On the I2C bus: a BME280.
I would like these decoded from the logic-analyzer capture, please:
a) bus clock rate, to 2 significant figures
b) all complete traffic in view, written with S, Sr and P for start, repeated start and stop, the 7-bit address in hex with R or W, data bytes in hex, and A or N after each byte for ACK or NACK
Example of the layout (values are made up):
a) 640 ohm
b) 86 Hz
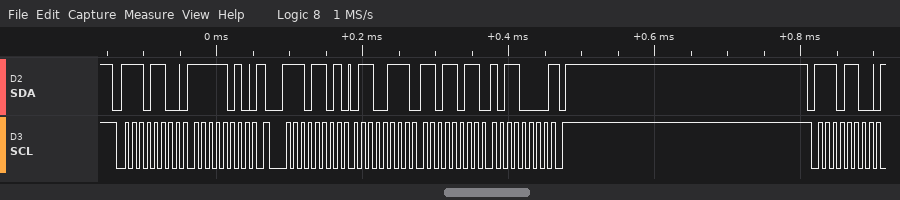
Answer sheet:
a) 100 kHz
b) S 76W A FA A Sr 76R A 67 A DB A B0 N P S 76W A
